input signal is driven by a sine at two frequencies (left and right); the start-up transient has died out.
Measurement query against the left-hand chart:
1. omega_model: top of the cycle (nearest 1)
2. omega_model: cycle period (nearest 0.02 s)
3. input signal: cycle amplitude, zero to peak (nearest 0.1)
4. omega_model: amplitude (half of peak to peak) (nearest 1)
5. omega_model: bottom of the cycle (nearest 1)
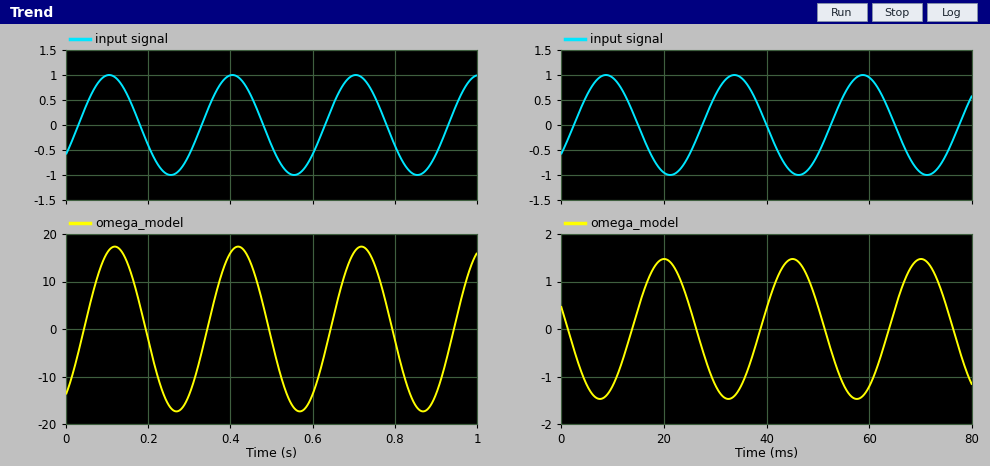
17
0.30 s
1.0
17
-17
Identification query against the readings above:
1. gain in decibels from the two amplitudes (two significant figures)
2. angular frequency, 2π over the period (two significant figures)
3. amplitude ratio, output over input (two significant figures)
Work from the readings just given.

25 dB
21 rad/s
17
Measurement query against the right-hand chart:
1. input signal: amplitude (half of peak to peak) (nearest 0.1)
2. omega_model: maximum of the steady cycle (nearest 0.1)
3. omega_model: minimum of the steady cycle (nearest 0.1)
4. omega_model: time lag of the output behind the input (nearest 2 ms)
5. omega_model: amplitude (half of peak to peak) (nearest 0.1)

1.0
1.5
-1.5
12 ms
1.5
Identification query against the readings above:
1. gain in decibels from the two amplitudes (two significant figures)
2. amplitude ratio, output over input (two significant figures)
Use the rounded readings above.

3.5 dB
1.5
